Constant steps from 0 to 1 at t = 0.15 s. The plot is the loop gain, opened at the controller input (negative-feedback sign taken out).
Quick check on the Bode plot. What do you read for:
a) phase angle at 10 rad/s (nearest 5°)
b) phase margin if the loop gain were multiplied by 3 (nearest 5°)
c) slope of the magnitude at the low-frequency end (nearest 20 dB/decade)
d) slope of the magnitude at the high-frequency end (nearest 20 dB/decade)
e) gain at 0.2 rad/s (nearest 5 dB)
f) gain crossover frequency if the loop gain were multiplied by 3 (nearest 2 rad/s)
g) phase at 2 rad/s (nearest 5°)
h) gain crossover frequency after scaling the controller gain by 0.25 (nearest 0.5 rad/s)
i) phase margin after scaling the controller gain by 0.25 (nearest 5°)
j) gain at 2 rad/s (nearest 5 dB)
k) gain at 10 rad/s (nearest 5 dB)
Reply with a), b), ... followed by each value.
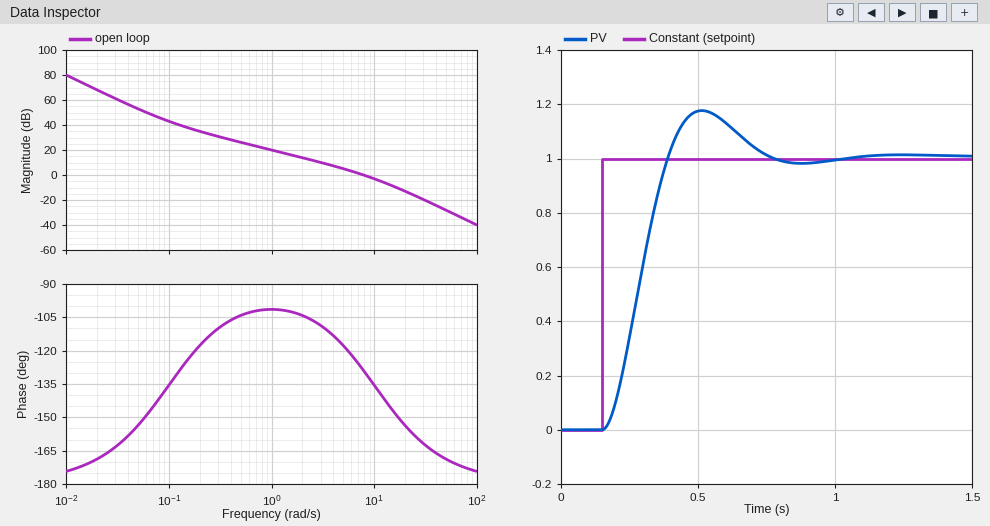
a) -135°
b) 30°
c) -40 dB/decade
d) -40 dB/decade
e) 35 dB
f) 16 rad/s
g) -105°
h) 2.5 rad/s
i) 75°
j) 15 dB
k) -5 dB
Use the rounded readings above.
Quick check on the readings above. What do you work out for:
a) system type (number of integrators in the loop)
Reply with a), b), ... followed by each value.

a) 2
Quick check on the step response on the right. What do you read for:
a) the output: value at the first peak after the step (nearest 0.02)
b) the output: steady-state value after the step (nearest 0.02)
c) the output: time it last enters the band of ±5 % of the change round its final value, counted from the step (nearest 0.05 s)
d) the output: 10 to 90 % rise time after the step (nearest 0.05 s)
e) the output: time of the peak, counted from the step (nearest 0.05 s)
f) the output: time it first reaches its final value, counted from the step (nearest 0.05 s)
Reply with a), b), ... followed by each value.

a) 1.18
b) 1.00
c) 0.55 s
d) 0.15 s
e) 0.35 s
f) 0.25 s
